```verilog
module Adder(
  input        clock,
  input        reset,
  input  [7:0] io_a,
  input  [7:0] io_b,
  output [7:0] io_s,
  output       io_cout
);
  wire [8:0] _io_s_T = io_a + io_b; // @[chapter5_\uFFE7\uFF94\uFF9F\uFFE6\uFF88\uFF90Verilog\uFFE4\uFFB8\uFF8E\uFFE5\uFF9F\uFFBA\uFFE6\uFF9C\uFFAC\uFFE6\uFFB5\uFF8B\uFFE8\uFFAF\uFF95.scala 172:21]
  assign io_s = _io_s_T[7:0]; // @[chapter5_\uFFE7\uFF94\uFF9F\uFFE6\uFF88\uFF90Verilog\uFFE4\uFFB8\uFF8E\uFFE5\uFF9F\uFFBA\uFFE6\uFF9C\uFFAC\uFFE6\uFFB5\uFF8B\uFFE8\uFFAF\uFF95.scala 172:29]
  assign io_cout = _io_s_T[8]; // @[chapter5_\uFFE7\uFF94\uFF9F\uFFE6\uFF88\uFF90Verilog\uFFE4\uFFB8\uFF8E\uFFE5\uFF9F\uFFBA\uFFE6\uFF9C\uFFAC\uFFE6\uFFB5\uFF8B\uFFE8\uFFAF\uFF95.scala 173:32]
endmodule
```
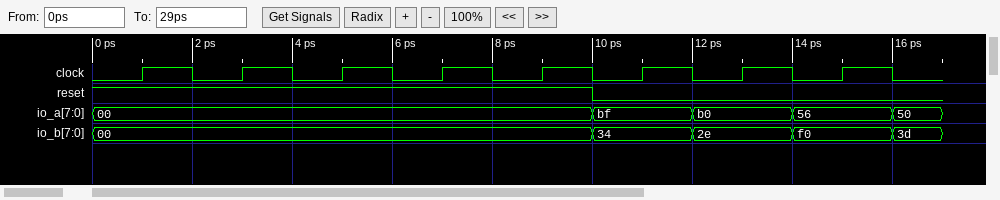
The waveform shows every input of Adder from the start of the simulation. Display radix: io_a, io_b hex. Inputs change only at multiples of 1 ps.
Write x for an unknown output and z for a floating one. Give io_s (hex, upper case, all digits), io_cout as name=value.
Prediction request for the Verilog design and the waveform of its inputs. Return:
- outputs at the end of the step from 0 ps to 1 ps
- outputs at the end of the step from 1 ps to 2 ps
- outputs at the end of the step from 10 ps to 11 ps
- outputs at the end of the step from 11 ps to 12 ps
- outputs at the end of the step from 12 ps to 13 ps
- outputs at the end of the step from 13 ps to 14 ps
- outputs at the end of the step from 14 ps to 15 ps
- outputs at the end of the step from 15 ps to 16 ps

io_s=00, io_cout=0
io_s=00, io_cout=0
io_s=F3, io_cout=0
io_s=F3, io_cout=0
io_s=DE, io_cout=0
io_s=DE, io_cout=0
io_s=46, io_cout=1
io_s=46, io_cout=1
